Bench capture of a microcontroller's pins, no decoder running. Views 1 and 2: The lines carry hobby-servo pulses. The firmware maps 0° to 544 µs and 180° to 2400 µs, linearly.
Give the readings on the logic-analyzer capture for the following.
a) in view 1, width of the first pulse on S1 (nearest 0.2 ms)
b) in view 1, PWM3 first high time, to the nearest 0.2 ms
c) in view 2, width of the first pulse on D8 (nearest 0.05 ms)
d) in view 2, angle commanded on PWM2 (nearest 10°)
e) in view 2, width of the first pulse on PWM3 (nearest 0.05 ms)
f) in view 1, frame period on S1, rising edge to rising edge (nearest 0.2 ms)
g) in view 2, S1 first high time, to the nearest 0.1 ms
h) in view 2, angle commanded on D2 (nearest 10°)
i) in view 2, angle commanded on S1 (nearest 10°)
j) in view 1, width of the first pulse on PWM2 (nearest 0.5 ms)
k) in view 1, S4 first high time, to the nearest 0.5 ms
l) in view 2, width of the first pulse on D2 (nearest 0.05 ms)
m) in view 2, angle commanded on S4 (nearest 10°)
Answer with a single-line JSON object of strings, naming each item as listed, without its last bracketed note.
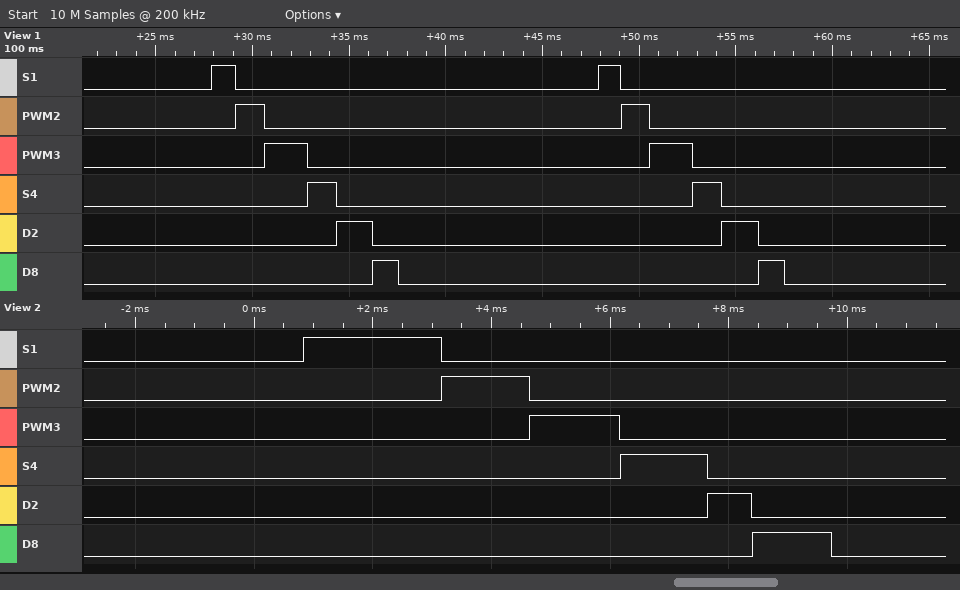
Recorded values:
{"in view 1, width of the first pulse on S1": "1.2 ms", "in view 1, PWM3 first high time, to the nearest 0.2 ms": "2.2 ms", "in view 2, width of the first pulse on D8": "1.35 ms", "in view 2, angle commanded on PWM2": "90°", "in view 2, width of the first pulse on PWM3": "1.50 ms", "in view 1, frame period on S1, rising edge to rising edge": "20.0 ms", "in view 2, S1 first high time, to the nearest 0.1 ms": "2.3 ms", "in view 2, angle commanded on D2": "20°", "in view 2, angle commanded on S1": "170°", "in view 1, width of the first pulse on PWM2": "1.5 ms", "in view 1, S4 first high time, to the nearest 0.5 ms": "1.5 ms", "in view 2, width of the first pulse on D2": "0.75 ms", "in view 2, angle commanded on S4": "90°"}
